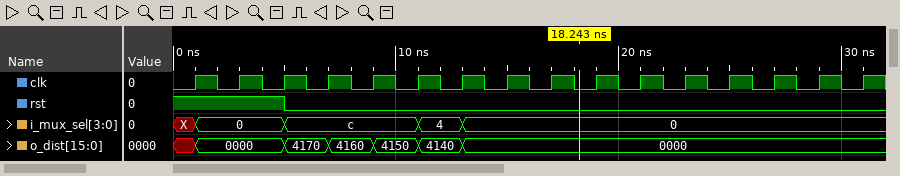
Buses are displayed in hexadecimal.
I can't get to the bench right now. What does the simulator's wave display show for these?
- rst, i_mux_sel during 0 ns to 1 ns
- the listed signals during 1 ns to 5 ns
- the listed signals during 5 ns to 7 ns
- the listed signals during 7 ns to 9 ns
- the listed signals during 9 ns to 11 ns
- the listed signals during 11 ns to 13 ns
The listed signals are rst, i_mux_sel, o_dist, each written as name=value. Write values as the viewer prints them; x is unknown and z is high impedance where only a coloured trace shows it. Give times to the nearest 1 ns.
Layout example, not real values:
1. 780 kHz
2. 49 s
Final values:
1. rst=1, i_mux_sel=X
2. rst=1, i_mux_sel=0, o_dist=0000
3. rst=0, i_mux_sel=c, o_dist=4170
4. rst=0, i_mux_sel=c, o_dist=4160
5. rst=0, i_mux_sel=c, o_dist=4150
6. rst=0, i_mux_sel=4, o_dist=4140
